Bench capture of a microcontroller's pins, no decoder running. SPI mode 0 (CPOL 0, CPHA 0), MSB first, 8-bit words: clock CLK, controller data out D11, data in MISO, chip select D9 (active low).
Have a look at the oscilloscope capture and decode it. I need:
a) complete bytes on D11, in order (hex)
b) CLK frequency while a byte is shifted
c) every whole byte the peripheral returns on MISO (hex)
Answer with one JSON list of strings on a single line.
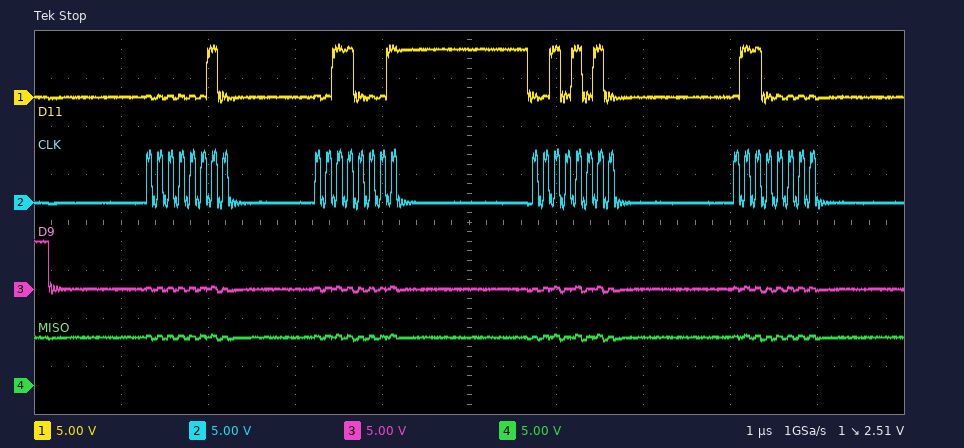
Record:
["02 31 2A 60", "8 MHz", "FF FF FF FF"]
